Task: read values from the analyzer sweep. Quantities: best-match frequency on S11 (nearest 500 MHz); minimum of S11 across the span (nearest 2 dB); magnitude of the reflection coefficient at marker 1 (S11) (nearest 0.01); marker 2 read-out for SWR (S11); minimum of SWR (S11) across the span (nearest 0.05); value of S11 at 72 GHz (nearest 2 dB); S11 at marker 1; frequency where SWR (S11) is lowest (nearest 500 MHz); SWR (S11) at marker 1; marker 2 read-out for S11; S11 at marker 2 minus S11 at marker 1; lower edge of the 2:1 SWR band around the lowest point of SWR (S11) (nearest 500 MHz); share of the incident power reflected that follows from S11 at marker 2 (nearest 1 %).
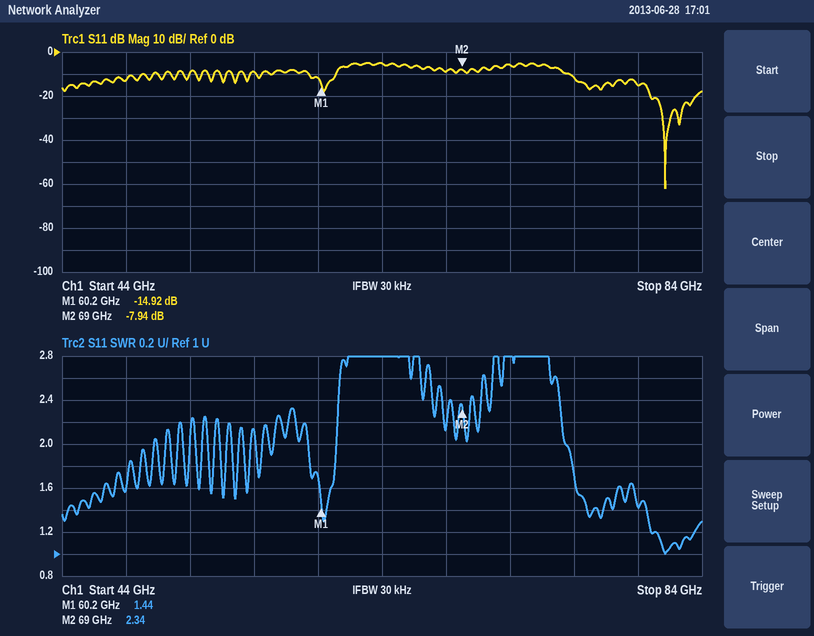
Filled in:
81.5 GHz
-62 dB
0.18
2.34
1.00
-6 dB
-14.92 dB
81.5 GHz
1.44
-7.94 dB
6.98 dB
75.5 GHz
16 %
